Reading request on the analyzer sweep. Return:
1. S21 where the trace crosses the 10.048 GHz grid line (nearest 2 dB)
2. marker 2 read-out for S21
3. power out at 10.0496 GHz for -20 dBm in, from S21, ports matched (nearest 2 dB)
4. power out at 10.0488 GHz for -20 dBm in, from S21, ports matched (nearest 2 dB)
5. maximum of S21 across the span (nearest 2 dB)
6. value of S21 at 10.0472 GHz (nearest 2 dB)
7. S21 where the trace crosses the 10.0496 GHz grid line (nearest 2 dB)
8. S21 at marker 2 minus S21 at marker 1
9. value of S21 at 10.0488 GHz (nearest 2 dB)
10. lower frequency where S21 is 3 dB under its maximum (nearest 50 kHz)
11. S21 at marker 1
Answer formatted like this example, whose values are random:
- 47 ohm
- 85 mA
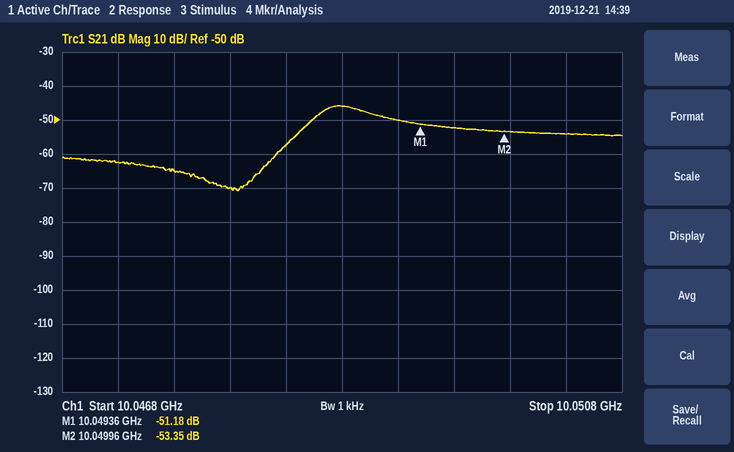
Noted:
- -70 dB
- -53.35 dB
- -72 dBm
- -66 dBm
- -46 dB
- -62 dB
- -52 dB
- -2.17 dB
- -46 dB
- 10.04860 GHz
- -51.18 dB
